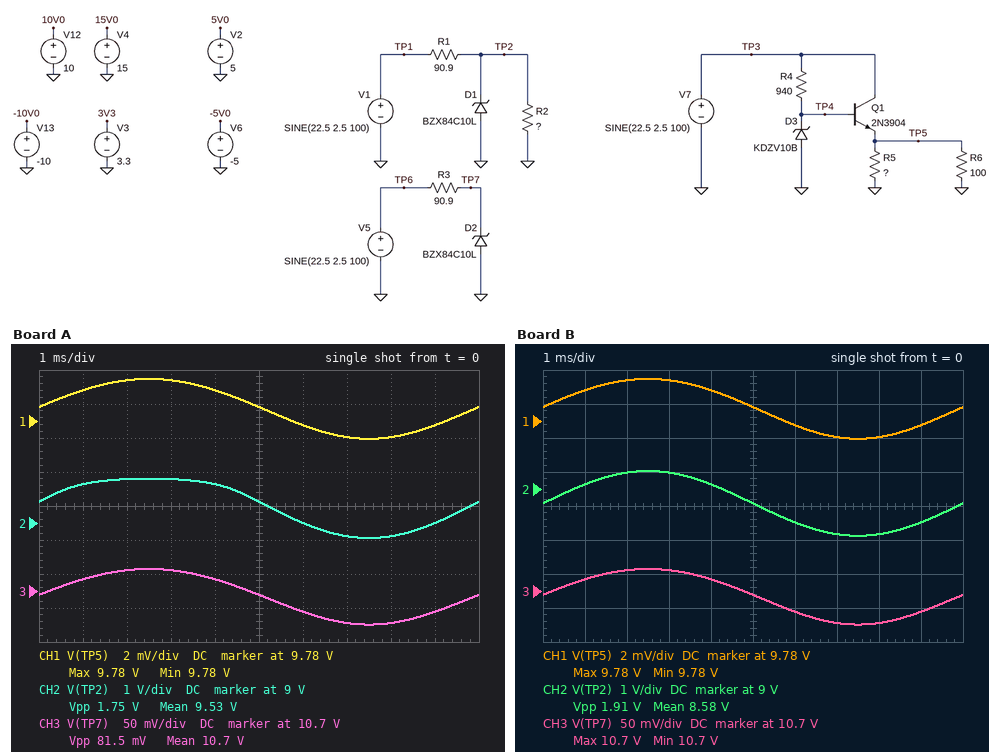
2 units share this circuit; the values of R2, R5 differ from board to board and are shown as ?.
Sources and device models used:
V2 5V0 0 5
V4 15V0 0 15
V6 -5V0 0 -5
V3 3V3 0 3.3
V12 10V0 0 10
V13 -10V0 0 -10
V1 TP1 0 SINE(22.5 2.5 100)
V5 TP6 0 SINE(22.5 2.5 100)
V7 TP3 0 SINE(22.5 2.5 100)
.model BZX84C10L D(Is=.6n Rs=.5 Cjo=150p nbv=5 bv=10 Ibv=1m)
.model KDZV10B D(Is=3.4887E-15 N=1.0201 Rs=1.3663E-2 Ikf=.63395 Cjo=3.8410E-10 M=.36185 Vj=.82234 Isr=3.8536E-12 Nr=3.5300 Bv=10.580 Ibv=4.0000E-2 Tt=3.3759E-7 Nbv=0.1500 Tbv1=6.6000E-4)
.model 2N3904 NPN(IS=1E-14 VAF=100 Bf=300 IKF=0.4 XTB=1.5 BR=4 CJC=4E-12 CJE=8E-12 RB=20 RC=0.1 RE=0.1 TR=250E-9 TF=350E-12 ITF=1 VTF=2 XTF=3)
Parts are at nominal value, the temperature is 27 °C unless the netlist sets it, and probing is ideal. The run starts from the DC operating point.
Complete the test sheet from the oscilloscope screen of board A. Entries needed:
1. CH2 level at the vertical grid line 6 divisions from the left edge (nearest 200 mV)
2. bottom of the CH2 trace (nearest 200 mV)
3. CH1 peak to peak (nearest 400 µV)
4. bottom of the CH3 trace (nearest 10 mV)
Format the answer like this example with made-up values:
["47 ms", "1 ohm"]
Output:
["9.0 V", "8.6 V", "3.6 mV", "10.65 V"]
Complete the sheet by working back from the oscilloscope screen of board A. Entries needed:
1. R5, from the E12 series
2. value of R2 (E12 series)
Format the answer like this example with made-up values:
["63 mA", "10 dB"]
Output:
["2.2 kΩ", "68 Ω"]
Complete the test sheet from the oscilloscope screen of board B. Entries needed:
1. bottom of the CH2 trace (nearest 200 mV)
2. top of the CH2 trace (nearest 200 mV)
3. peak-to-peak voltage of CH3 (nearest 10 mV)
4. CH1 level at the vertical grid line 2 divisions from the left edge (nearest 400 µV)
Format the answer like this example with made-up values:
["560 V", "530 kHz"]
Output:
["7.6 V", "9.6 V", "80 mV", "9.7824 V"]
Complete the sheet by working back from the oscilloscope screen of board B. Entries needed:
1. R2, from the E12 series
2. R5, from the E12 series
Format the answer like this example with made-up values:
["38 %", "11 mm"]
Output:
["56 Ω", "2.2 kΩ"]
